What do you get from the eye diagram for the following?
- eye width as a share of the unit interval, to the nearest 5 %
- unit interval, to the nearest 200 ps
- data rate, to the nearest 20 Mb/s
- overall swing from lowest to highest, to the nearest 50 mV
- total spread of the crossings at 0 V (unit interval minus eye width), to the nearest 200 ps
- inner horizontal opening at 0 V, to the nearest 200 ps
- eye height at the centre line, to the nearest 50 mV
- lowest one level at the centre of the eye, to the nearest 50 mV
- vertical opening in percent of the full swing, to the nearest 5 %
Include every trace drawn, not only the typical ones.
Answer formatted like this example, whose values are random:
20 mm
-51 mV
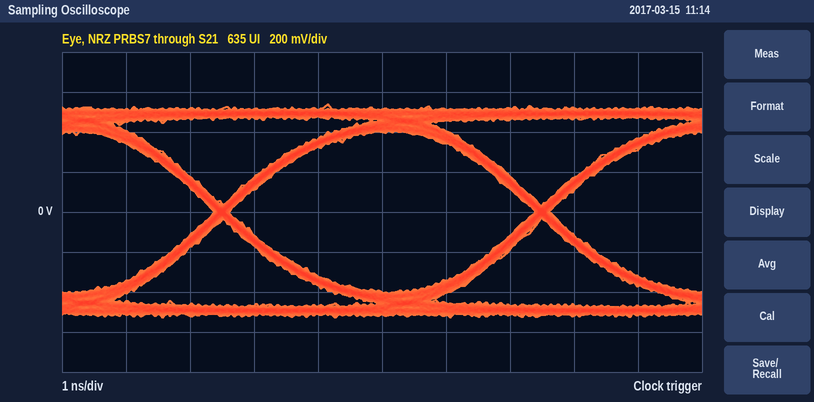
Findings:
95 %
5.0 ns
200 Mb/s
1.05 V
200 ps
4.8 ns
800 mV
400 mV
75 %
